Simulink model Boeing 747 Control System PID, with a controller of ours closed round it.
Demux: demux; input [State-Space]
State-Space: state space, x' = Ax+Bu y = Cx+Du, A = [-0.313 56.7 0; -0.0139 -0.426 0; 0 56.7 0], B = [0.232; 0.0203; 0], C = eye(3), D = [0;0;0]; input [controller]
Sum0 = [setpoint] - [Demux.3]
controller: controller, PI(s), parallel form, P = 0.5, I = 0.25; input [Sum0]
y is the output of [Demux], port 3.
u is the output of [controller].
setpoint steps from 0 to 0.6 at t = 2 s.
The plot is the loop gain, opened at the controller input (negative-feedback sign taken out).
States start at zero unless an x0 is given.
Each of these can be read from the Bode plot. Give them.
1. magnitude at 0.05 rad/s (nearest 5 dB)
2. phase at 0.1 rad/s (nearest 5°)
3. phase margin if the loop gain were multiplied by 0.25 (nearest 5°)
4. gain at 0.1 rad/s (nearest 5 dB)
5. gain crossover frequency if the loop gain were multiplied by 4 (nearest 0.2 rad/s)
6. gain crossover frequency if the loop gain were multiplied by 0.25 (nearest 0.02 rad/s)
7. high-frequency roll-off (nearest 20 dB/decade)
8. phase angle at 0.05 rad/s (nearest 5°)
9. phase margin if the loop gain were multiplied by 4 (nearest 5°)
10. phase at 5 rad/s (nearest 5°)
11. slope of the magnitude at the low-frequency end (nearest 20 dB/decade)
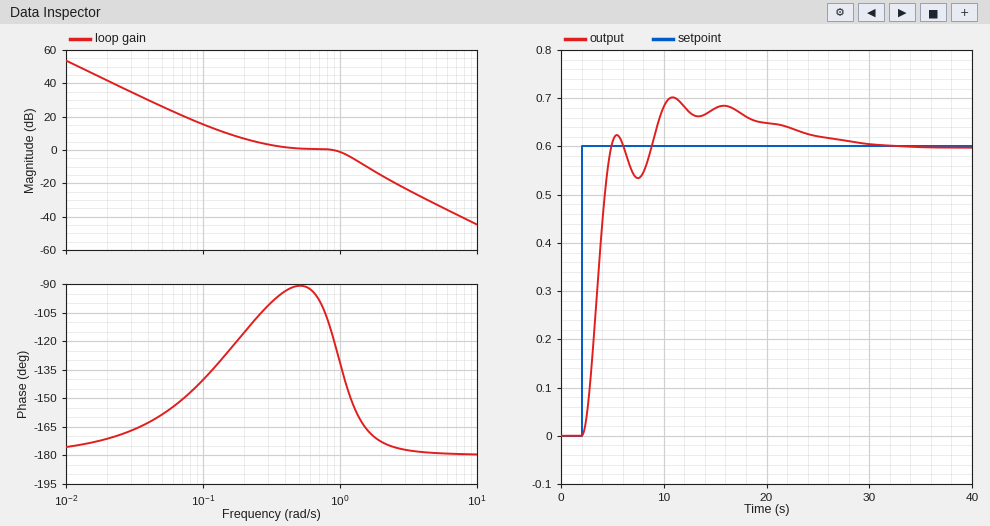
25 dB
-140°
50°
15 dB
1.8 rad/s
0.12 rad/s
-40 dB/decade
-160°
10°
-180°
-40 dB/decade
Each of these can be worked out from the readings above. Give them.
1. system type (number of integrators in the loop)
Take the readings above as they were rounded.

2
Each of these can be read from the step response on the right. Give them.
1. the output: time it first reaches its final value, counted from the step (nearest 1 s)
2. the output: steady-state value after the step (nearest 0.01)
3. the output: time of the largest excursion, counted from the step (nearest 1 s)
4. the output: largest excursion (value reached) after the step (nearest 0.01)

3 s
0.60
9 s
0.70
